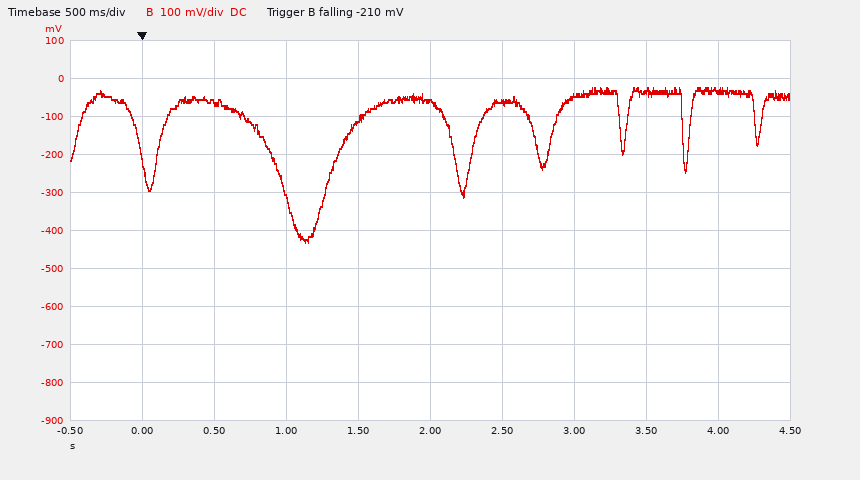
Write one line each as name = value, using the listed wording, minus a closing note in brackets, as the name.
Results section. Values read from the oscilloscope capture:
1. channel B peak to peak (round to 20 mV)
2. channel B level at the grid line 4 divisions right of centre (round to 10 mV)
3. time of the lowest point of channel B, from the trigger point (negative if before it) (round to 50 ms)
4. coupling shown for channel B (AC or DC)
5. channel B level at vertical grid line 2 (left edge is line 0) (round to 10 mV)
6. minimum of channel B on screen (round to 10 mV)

channel B peak to peak = 400 mV
channel B level at the grid line 4 divisions right of centre = -30 mV
time of the lowest point of channel B, from the trigger point (negative if before it) = +1.15 s
coupling shown for channel B = DC
channel B level at vertical grid line 2 (left edge is line 0) = -60 mV
minimum of channel B on screen = -430 mV
